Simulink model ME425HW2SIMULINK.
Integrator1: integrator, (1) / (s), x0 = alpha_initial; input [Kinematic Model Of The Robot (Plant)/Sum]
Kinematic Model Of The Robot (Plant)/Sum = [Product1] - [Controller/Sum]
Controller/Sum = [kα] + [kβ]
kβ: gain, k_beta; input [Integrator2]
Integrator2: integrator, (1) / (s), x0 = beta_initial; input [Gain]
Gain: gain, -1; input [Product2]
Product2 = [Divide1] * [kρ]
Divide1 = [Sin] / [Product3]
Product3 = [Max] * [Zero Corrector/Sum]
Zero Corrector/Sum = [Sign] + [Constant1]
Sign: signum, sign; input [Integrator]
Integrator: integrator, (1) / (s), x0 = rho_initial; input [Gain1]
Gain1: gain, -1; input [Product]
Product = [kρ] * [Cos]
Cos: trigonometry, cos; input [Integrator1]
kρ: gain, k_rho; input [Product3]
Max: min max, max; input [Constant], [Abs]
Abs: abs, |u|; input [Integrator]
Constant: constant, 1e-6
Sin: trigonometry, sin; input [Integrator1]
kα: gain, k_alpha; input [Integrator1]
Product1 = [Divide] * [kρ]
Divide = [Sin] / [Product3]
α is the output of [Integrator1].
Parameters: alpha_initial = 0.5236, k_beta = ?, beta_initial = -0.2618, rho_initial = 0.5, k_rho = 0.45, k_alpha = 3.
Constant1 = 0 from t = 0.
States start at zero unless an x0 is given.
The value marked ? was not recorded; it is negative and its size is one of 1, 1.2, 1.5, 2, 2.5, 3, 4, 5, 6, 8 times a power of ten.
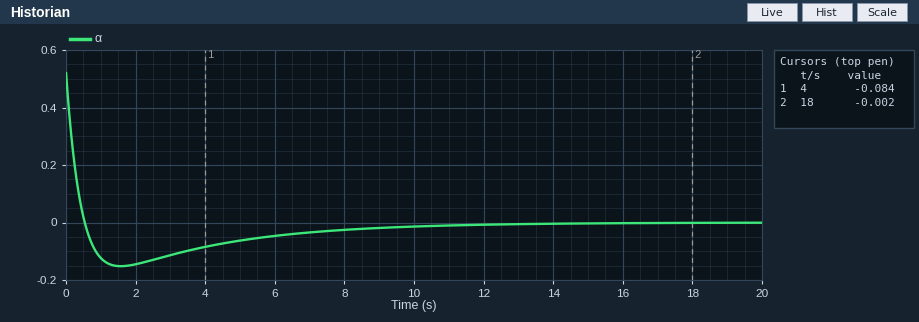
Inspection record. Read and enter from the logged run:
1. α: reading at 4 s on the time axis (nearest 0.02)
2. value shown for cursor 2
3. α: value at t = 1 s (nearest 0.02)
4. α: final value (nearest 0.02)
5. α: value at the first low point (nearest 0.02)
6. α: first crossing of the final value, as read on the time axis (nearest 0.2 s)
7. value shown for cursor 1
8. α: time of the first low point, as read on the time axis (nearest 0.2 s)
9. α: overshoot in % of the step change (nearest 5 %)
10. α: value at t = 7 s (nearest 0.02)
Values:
-0.08
-0.002
-0.12
0.00
-0.16
0.6 s
-0.084
1.6 s
30 %
-0.04
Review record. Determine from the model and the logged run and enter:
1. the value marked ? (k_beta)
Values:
-1.5
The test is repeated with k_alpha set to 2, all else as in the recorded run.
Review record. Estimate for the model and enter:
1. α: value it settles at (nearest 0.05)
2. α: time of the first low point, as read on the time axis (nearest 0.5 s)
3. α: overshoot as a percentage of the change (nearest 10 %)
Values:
0.00
2.0 s
40 %
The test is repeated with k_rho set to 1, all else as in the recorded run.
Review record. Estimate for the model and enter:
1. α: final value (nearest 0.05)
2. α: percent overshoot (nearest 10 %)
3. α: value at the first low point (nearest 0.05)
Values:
0.00
40 %
-0.20
